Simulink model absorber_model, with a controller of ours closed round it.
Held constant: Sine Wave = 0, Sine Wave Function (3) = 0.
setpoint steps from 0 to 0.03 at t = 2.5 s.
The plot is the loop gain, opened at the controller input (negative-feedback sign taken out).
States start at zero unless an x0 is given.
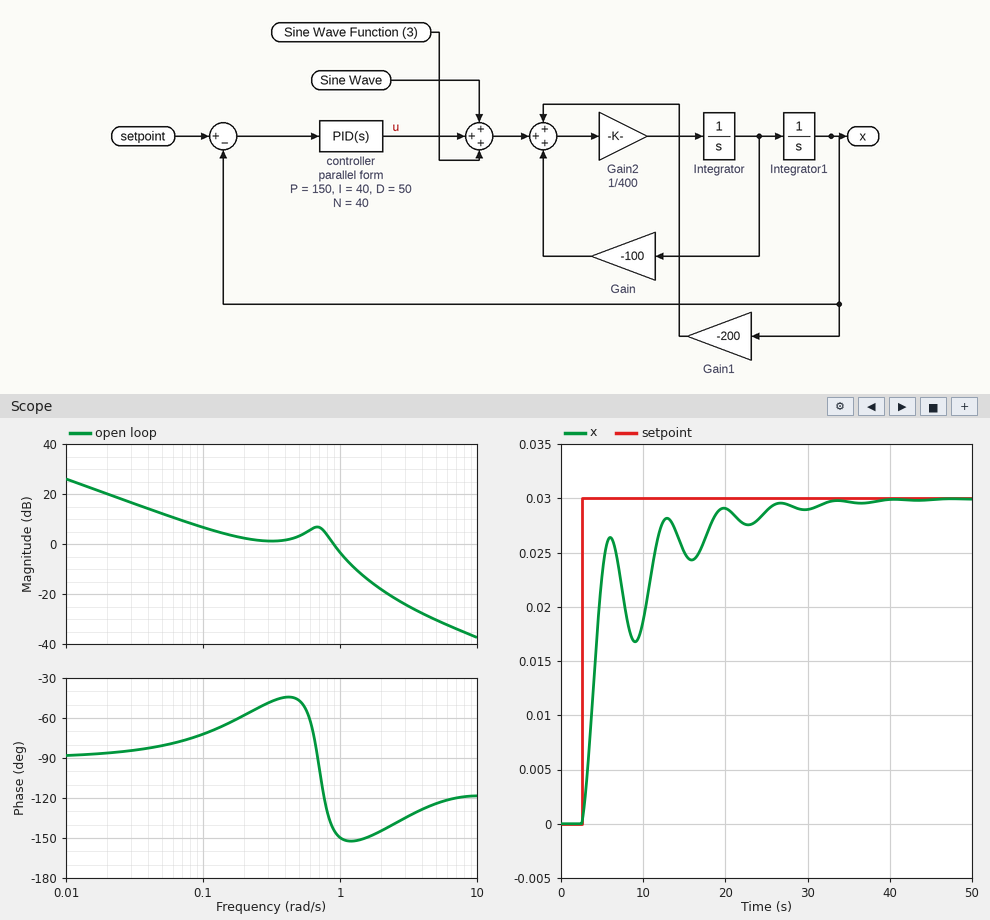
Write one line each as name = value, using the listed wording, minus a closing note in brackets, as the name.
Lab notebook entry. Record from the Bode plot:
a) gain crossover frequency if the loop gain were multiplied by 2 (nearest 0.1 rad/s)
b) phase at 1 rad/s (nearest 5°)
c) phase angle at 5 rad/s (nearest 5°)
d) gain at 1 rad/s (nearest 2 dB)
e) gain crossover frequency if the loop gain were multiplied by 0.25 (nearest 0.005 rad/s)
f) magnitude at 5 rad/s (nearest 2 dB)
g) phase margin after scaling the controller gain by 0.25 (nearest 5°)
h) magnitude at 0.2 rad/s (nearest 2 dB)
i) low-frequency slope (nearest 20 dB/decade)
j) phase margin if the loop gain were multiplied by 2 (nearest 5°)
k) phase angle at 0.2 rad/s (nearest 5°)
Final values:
gain crossover frequency if the loop gain were multiplied by 2 = 1.1 rad/s
phase at 1 rad/s = -150°
phase angle at 5 rad/s = -125°
gain at 1 rad/s = -4 dB
gain crossover frequency if the loop gain were multiplied by 0.25 = 0.050 rad/s
magnitude at 5 rad/s = -30 dB
phase margin after scaling the controller gain by 0.25 = 100°
magnitude at 0.2 rad/s = 2 dB
low-frequency slope = -20 dB/decade
phase margin if the loop gain were multiplied by 2 = 30°
phase angle at 0.2 rad/s = -60°
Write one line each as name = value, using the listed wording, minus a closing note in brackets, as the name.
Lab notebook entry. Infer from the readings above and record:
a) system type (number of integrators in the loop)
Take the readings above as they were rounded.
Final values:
system type = 1
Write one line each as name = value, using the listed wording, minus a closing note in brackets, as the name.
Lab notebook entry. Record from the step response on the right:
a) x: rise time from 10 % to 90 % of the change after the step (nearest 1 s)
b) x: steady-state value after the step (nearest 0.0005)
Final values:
x: rise time from 10 % to 90 % of the change after the step = 9 s
x: steady-state value after the step = 0.0300
